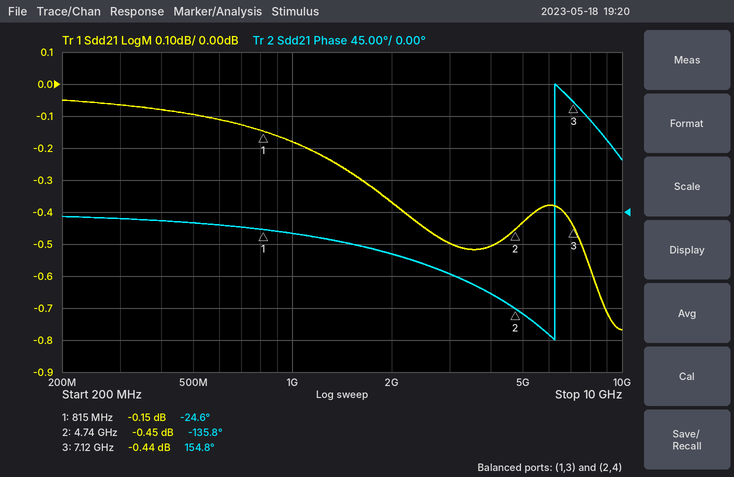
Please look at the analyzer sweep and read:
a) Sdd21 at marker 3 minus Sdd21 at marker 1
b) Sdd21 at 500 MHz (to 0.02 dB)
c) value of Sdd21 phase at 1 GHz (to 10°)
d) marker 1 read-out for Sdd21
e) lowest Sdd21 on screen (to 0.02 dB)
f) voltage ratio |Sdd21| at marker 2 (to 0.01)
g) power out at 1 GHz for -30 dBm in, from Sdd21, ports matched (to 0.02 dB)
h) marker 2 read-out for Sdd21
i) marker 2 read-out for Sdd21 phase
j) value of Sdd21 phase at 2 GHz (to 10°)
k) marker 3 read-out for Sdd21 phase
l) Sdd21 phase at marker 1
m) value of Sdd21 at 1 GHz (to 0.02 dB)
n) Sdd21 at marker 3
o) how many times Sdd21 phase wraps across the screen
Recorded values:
-0.29 dB
-0.10 dB
-30°
-0.15 dB
-0.76 dB
0.95
-30.18 dBm
-0.45 dB
-135.8°
-60°
154.8°
-24.6°
-0.18 dB
-0.44 dB
1
